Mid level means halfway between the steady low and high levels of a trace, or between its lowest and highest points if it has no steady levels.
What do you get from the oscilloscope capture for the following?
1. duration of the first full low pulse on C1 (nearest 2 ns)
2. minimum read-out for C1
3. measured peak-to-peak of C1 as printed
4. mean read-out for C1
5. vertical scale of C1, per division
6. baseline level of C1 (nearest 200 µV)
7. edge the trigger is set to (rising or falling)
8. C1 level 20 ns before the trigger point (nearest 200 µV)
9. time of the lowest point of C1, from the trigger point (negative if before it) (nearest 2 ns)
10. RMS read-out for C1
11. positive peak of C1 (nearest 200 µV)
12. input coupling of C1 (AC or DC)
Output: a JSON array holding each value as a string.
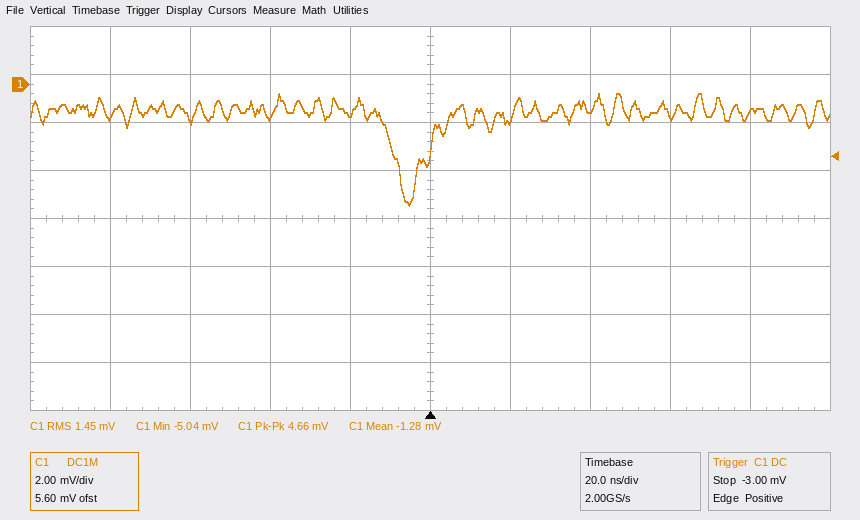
["10 ns", "-5.04 mV", "4.66 mV", "-1.28 mV", "2 mV", "-1.2 mV", "rising", "-1.2 mV", "-6 ns", "1.45 mV", "-400 µV", "DC"]
